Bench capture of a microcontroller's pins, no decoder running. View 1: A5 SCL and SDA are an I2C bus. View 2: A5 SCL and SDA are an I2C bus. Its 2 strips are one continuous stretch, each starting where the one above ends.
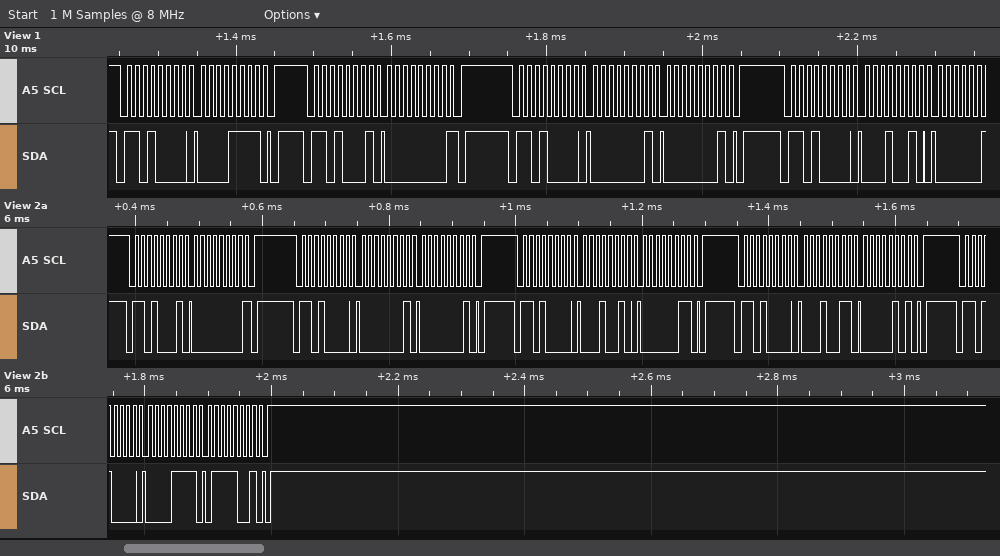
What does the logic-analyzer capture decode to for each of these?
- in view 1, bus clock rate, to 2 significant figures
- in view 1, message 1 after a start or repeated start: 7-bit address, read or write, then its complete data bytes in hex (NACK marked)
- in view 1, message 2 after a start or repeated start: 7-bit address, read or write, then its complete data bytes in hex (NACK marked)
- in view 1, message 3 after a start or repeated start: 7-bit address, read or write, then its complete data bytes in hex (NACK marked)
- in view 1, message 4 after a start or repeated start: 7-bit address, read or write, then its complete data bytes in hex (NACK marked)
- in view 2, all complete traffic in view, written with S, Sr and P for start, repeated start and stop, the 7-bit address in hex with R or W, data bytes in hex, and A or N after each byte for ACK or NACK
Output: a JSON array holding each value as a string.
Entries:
["100 kHz", "0x68 write: 0F", "0x68 read: 00 NACK", "0x68 write: 01 01", "0x68 write: 12", "S 68R A 00 N P S 68W A 01 A 01 A P S 68W A 12 A 03 A P S 68W A 13 A 05 A P S 68W A 0F A 79 A P"]
